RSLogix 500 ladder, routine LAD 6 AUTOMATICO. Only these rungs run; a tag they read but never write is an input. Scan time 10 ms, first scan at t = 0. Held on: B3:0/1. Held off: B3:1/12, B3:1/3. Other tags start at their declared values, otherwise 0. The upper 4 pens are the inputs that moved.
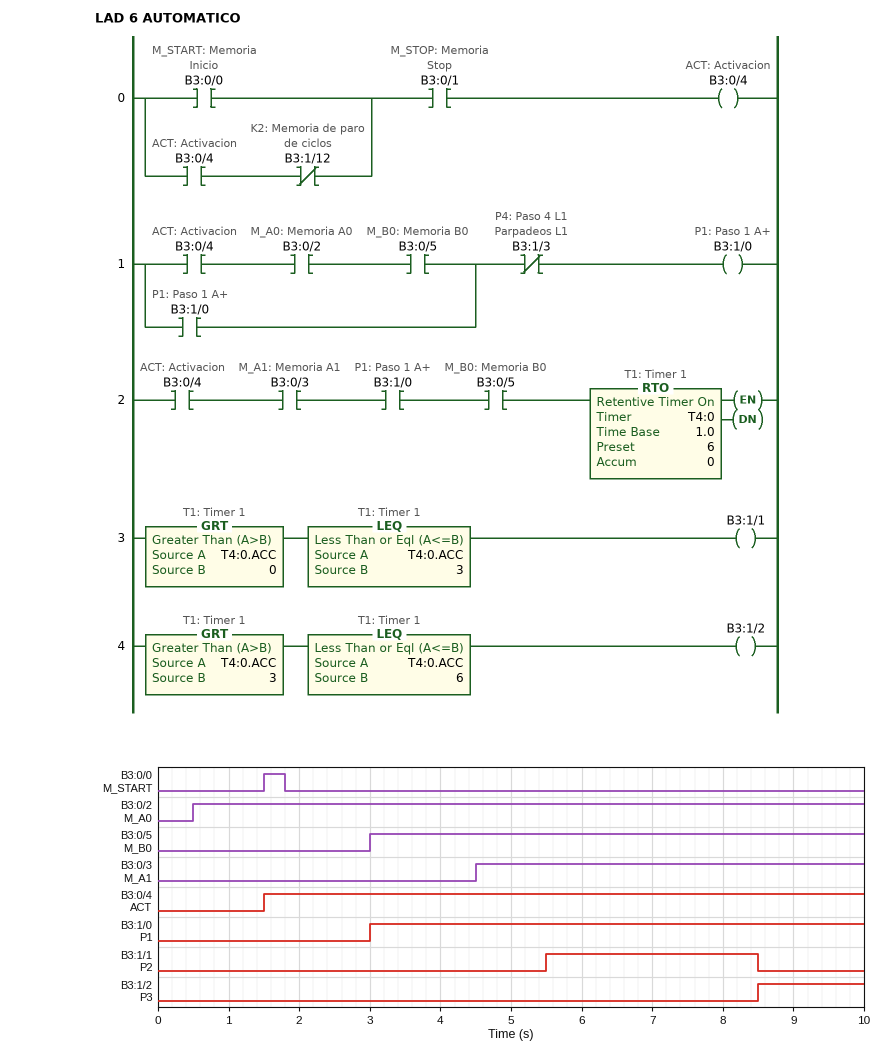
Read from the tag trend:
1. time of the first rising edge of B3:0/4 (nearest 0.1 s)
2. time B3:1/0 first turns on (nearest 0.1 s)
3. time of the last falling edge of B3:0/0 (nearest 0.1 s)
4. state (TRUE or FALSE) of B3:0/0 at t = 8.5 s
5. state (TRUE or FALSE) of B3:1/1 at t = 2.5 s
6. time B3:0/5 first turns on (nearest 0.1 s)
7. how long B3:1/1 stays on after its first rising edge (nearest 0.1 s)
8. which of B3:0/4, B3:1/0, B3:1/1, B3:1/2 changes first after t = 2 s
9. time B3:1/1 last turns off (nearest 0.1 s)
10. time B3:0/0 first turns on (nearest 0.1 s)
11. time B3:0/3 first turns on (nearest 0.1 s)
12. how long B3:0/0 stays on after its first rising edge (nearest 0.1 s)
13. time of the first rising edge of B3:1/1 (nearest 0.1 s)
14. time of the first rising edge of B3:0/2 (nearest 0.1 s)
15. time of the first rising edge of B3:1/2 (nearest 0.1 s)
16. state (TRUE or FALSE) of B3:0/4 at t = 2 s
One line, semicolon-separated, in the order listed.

1.5 s; 3.0 s; 1.8 s; FALSE; FALSE; 3.0 s; 3.0 s; B3:1/0; 8.5 s; 1.5 s; 4.5 s; 0.3 s; 5.5 s; 0.5 s; 8.5 s; TRUE
